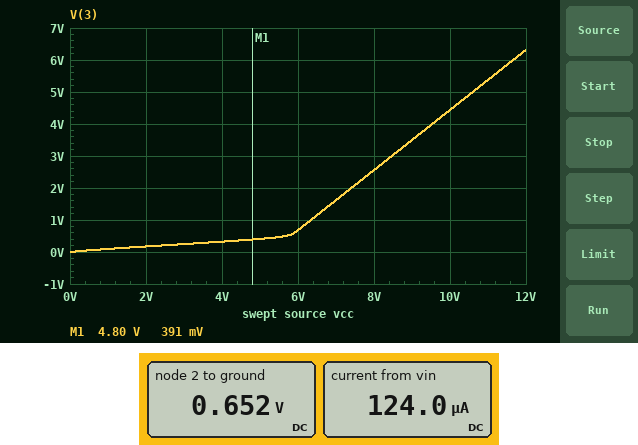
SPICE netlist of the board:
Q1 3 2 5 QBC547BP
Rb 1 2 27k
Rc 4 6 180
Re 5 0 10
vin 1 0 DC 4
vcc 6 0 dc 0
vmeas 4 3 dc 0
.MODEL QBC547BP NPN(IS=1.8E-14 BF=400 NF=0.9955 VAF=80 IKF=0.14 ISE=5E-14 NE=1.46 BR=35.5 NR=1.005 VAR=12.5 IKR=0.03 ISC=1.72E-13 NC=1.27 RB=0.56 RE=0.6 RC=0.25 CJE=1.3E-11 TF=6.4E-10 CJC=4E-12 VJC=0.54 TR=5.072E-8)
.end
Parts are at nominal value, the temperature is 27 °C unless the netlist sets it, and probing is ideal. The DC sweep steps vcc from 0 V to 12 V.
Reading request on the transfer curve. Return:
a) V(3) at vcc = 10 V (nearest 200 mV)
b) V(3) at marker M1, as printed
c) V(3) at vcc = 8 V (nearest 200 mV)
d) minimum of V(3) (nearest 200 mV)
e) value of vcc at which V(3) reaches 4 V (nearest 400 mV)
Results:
4.4 V
391 mV
2.6 V
0 V
9.6 V
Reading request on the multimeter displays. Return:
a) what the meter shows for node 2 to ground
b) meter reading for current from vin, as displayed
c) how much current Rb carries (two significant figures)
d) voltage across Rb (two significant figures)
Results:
0.652 V
124.0 µA
120 µA
3.3 V
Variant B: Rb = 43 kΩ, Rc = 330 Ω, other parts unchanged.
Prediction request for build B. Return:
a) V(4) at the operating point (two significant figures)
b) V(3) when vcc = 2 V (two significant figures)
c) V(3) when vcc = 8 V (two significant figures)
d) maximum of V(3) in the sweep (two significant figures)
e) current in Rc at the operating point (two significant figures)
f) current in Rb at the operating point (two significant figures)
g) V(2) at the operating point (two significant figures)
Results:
-2.6 mV
120 mV
1.3 V
5.0 V
7.9 µA
78 µA
640 mV
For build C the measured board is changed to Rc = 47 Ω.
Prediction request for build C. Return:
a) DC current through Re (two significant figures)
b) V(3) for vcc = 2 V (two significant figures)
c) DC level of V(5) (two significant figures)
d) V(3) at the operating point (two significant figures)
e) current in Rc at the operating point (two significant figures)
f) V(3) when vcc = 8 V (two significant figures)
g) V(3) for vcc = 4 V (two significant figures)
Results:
160 µA
610 mV
1.6 mV
-1.7 mV
36 µA
6.5 V
2.6 V
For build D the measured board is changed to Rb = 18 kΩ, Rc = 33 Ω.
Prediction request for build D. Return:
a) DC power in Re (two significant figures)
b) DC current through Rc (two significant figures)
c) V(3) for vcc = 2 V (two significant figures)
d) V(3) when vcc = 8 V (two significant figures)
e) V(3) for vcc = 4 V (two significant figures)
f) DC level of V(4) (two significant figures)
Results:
510 nW
40 µA
680 mV
6.6 V
2.6 V
-1.3 mV
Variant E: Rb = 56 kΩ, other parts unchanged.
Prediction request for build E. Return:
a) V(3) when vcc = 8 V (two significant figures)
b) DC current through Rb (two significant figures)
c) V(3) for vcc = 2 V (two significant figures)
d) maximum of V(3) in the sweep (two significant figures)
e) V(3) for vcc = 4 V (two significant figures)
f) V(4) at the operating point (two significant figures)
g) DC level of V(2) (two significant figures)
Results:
5.0 V
60 µA
210 mV
8.8 V
1.1 V
-2.3 mV
630 mV
